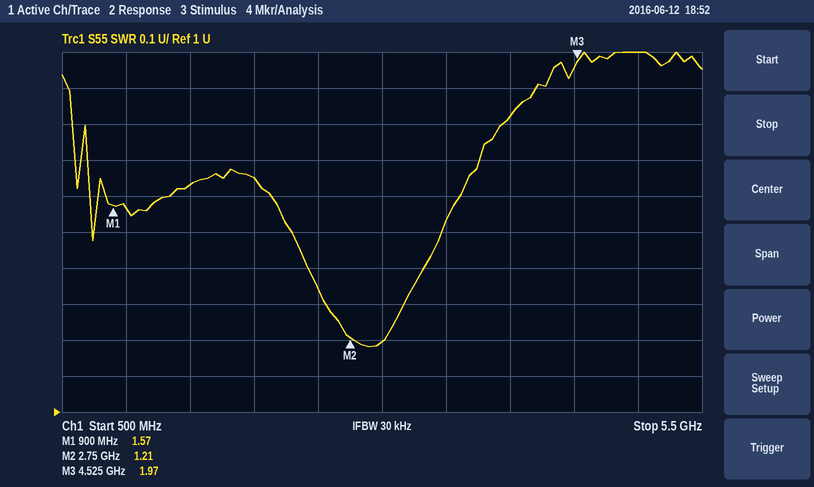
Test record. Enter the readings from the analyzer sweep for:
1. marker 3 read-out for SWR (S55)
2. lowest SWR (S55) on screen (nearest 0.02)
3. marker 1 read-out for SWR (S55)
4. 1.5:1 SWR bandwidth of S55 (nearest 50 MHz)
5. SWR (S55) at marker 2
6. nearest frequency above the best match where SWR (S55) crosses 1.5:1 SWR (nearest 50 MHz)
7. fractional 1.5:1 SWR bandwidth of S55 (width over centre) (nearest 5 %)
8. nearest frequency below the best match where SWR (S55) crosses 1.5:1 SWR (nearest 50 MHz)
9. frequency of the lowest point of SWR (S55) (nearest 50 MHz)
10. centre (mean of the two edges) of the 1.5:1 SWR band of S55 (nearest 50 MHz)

1.97
1.18
1.57
1.15 GHz
1.21
3.45 GHz
40 %
2.30 GHz
2.90 GHz
2.90 GHz
